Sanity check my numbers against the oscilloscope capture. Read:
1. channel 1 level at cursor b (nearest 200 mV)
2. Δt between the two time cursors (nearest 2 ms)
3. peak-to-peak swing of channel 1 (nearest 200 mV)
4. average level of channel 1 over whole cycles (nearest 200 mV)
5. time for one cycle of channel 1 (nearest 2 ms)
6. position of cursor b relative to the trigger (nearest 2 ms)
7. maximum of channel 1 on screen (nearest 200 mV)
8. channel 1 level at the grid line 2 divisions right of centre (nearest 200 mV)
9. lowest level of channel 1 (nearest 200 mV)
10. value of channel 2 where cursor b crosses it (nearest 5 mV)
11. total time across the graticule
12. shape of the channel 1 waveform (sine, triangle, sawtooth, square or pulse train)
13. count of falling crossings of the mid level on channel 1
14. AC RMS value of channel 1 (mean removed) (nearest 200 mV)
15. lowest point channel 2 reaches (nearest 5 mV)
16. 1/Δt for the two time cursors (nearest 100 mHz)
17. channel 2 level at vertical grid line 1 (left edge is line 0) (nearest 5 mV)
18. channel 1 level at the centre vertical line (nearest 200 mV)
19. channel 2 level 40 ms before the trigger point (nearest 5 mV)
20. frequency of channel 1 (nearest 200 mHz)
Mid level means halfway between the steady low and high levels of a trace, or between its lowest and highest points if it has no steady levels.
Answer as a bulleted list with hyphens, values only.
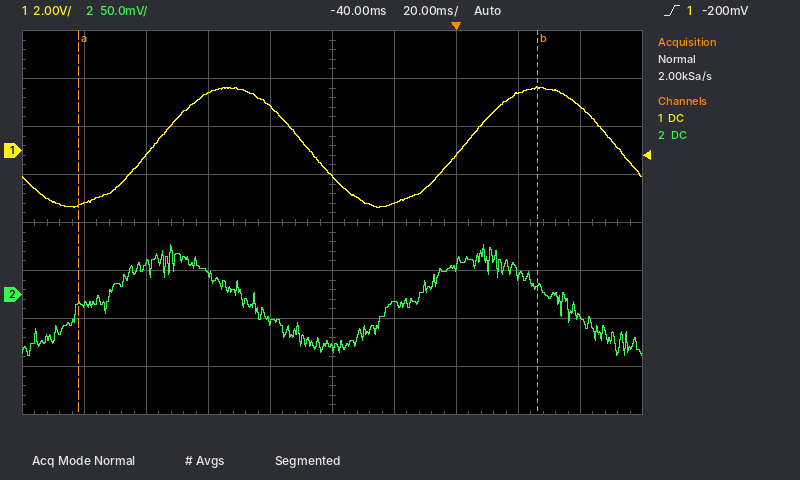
- 2.6 V
- 148 ms
- 5.0 V
- 200 mV
- 100 ms
- +26 ms
- 2.6 V
- -200 mV
- -2.4 V
- 10 mV
- 200 ms
- sine
- 2
- 1.8 V
- -65 mV
- 6.8 Hz
- -10 mV
- -1.0 V
- -55 mV
- 10.0 Hz
